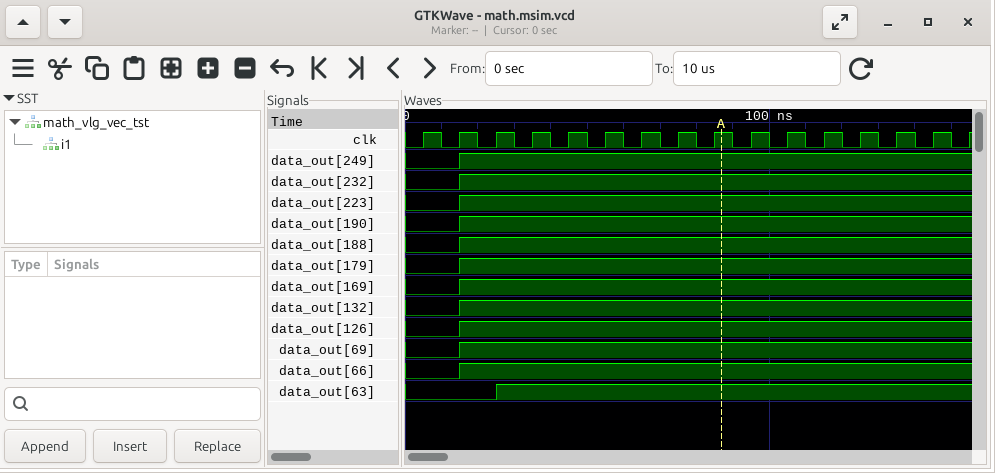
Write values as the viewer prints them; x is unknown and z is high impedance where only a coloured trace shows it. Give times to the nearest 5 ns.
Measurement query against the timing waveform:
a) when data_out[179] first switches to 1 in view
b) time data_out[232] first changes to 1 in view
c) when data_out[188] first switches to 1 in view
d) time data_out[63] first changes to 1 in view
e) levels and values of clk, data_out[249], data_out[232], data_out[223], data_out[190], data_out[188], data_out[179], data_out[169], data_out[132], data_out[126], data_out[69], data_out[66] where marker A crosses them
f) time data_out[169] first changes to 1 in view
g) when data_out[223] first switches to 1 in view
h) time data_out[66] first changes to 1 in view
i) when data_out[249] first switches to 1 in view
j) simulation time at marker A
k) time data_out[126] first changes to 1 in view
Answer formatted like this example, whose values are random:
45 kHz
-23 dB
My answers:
15 ns
15 ns
15 ns
25 ns
clk=1, data_out[249]=1, data_out[232]=1, data_out[223]=1, data_out[190]=1, data_out[188]=1, data_out[179]=1, data_out[169]=1, data_out[132]=1, data_out[126]=1, data_out[69]=1, data_out[66]=1
15 ns
15 ns
15 ns
15 ns
85 ns
15 ns
